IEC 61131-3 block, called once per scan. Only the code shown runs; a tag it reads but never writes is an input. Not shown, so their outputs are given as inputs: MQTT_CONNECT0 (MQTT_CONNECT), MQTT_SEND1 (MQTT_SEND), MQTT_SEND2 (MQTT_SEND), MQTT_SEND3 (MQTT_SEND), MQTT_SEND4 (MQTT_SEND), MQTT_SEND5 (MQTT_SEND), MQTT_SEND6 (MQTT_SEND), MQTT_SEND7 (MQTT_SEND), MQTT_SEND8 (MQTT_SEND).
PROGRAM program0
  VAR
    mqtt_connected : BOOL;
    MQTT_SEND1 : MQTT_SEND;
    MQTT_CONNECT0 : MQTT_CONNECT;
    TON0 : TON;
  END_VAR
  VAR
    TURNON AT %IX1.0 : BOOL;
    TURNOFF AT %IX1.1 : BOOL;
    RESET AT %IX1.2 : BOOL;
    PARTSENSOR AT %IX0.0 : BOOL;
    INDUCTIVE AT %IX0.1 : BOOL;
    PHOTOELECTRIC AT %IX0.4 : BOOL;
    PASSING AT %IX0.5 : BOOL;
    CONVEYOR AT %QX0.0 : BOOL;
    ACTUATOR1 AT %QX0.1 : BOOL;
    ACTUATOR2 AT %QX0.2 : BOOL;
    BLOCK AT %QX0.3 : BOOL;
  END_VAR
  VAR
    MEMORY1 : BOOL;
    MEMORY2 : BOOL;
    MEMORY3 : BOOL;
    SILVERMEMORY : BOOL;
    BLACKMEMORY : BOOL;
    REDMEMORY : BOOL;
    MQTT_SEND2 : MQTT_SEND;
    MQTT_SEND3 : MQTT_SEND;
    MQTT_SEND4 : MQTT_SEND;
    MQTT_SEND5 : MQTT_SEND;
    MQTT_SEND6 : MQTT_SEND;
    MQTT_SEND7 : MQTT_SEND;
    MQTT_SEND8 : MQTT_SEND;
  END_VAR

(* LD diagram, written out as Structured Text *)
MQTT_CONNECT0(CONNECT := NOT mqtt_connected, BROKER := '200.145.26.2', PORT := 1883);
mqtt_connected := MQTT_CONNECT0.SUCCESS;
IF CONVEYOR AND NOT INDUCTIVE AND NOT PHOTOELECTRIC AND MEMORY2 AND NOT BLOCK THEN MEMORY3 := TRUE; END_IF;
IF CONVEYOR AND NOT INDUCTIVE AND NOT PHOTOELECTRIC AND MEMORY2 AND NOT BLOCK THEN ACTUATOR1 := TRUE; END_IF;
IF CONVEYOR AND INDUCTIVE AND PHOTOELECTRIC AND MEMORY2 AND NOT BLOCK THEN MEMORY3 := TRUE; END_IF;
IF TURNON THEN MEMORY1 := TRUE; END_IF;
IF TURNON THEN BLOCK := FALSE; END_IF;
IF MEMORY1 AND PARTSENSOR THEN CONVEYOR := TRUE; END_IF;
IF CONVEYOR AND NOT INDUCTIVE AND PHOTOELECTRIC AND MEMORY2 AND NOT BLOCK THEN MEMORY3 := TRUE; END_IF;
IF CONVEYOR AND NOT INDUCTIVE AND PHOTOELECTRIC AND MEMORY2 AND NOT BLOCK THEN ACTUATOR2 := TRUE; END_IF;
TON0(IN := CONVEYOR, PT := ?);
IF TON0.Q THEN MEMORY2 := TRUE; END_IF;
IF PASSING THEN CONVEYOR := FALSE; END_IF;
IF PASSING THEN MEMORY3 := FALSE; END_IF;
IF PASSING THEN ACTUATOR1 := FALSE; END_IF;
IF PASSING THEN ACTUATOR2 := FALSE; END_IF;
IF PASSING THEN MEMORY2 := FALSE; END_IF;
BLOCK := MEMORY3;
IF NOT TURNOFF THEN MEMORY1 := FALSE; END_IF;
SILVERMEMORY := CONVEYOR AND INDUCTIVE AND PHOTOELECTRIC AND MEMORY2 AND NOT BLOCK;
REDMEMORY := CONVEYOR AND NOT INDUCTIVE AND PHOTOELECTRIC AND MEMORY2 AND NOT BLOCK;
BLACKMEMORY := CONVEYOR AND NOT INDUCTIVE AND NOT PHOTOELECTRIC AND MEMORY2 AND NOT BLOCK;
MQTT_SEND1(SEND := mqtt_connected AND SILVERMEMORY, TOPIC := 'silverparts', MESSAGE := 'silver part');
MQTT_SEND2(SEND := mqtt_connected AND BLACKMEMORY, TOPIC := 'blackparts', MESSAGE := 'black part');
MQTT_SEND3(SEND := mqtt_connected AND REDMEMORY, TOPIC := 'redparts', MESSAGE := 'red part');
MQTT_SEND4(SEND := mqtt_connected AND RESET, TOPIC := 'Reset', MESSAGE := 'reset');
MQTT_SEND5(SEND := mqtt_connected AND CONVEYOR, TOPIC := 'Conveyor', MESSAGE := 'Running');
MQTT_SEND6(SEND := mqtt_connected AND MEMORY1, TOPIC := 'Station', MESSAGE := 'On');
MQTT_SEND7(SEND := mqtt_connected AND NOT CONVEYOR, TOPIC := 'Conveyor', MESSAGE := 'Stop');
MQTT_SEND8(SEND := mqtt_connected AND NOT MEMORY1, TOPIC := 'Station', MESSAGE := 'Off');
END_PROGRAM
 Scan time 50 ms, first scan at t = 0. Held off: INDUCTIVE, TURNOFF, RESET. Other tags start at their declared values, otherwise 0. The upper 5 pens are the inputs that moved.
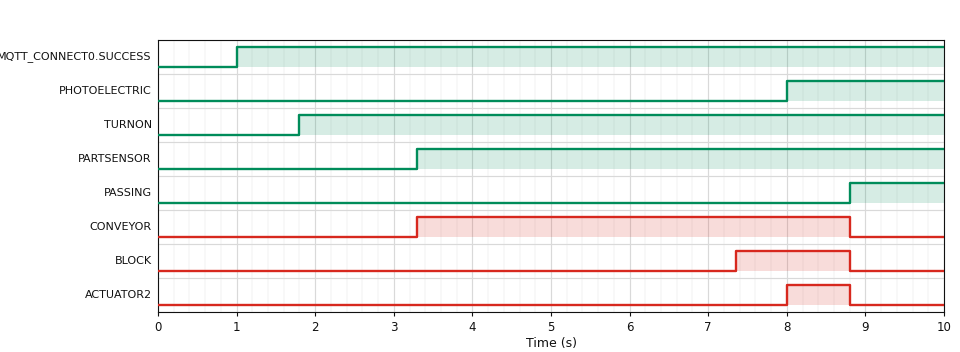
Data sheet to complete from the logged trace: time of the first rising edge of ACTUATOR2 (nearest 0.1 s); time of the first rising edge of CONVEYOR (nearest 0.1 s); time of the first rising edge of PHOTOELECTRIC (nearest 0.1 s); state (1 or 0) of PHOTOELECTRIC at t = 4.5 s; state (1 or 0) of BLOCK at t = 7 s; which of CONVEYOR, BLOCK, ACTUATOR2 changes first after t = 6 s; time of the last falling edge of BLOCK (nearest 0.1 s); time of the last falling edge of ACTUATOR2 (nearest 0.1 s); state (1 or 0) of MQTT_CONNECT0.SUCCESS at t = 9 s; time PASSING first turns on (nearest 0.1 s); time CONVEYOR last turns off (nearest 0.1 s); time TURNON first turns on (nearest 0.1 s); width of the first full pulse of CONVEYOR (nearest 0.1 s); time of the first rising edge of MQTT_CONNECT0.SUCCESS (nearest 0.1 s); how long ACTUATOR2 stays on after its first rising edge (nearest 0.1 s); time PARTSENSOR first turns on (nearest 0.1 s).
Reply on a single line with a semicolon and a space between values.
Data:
8.0 s; 3.3 s; 8.0 s; 0; 0; BLOCK; 8.8 s; 8.8 s; 1; 8.8 s; 8.8 s; 1.8 s; 5.5 s; 1.0 s; 0.8 s; 3.3 s
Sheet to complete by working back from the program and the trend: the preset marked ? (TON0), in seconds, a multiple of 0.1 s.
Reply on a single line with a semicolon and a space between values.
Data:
4.0 s
